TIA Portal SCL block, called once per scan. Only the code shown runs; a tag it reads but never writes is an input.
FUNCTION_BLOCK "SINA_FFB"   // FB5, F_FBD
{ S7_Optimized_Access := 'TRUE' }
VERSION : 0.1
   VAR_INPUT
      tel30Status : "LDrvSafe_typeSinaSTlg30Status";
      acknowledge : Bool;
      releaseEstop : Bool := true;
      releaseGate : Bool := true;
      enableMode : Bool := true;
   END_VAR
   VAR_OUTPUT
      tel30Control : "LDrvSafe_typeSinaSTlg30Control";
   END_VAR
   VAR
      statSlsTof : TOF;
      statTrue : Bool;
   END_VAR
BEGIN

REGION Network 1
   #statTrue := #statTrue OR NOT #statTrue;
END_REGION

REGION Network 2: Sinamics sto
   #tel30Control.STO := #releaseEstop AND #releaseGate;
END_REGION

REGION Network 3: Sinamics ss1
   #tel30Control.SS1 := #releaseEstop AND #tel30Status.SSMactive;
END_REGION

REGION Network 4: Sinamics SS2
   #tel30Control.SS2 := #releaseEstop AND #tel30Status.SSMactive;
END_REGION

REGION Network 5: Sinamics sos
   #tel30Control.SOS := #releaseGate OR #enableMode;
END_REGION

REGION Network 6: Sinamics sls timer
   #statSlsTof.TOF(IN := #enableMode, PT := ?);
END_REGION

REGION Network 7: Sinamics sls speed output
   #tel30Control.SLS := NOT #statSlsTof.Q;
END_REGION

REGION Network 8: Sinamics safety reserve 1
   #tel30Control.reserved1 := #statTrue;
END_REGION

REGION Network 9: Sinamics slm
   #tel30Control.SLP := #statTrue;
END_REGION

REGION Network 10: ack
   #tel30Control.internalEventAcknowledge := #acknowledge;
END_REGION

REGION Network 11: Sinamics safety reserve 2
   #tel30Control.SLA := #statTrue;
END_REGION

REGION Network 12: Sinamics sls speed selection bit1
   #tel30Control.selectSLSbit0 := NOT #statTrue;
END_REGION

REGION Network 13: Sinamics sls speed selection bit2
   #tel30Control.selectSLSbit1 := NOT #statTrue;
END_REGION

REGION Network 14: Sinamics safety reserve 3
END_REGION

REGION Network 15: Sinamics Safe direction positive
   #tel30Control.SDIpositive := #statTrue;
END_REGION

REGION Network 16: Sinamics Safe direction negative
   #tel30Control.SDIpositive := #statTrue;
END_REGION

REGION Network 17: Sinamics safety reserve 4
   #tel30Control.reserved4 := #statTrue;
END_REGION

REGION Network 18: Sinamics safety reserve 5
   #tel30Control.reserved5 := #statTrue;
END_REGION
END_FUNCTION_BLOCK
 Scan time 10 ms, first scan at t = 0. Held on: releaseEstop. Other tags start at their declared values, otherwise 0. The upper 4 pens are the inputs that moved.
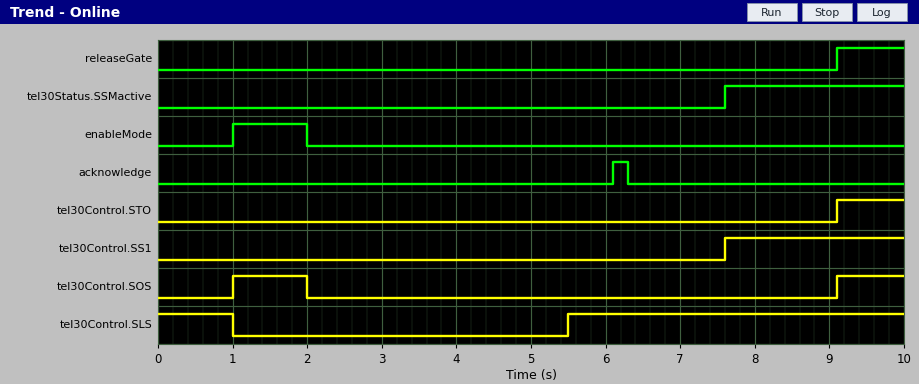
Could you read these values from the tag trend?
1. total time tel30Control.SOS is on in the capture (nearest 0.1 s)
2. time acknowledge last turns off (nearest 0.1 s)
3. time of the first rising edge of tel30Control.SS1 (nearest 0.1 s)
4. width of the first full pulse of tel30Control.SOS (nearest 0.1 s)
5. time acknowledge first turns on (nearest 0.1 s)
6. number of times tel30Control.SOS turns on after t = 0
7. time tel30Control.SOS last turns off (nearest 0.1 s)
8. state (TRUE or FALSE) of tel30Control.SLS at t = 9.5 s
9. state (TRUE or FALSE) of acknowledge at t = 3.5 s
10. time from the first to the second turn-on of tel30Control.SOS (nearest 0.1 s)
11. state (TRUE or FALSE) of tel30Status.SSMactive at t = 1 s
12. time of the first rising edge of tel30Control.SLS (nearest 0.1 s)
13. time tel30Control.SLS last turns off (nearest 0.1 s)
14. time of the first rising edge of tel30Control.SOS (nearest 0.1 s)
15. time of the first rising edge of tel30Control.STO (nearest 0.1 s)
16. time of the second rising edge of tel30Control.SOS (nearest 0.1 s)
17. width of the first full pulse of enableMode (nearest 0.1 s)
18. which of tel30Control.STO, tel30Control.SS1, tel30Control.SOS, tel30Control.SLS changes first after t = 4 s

1.9 s
6.3 s
7.6 s
1.0 s
6.1 s
2
2.0 s
TRUE
FALSE
8.1 s
FALSE
5.5 s
1.0 s
1.0 s
9.1 s
9.1 s
1.0 s
tel30Control.SLS
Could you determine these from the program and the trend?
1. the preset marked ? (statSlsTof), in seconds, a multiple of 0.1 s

3.5 s
